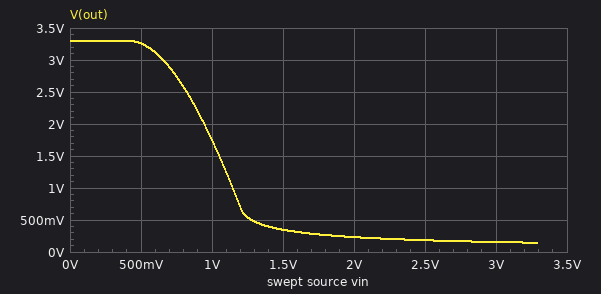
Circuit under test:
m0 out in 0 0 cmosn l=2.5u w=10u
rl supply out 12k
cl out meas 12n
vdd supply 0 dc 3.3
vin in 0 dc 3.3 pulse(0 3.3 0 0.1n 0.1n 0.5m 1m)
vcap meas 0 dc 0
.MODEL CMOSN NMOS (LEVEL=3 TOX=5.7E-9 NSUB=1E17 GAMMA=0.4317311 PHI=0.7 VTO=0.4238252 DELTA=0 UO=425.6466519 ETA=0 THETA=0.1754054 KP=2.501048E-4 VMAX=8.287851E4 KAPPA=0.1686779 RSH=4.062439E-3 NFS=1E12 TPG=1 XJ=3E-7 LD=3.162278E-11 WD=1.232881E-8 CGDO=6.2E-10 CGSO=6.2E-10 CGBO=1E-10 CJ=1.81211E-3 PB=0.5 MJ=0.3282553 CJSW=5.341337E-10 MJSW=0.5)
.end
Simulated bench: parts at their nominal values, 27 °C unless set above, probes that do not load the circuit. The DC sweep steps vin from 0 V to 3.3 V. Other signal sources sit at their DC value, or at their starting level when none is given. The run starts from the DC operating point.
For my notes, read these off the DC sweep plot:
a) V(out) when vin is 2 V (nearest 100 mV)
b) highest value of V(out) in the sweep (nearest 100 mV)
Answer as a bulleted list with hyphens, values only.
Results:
- 200 mV
- 3.3 V
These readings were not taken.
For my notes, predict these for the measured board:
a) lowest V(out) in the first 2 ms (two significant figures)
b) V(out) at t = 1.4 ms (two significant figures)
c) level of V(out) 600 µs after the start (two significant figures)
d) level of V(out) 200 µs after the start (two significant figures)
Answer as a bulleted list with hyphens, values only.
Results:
- 140 mV
- 140 mV
- 1.7 V
- 140 mV
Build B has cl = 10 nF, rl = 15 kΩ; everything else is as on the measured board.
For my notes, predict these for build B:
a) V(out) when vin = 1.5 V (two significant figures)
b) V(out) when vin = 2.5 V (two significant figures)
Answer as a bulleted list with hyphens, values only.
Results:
- 270 mV
- 150 mV
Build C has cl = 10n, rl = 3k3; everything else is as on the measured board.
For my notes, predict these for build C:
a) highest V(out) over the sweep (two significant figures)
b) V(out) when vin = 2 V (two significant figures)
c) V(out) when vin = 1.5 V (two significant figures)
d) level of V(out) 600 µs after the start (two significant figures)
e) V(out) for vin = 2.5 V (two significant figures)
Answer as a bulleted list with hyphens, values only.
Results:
- 3.3 V
- 1.0 V
- 2.0 V
- 3.2 V
- 700 mV
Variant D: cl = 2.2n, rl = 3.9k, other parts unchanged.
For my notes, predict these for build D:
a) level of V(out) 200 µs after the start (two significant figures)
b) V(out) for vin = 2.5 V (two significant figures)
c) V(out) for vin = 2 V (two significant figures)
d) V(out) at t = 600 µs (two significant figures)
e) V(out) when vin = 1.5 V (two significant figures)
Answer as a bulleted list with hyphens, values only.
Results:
- 440 mV
- 590 mV
- 820 mV
- 3.3 V
- 1.8 V
